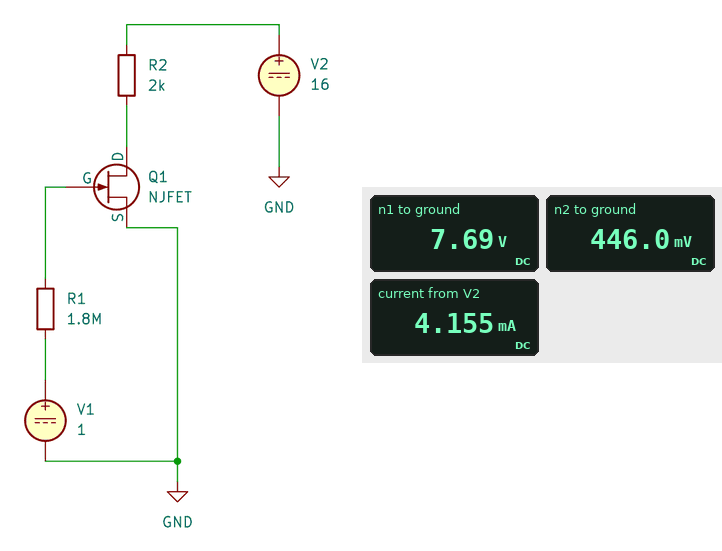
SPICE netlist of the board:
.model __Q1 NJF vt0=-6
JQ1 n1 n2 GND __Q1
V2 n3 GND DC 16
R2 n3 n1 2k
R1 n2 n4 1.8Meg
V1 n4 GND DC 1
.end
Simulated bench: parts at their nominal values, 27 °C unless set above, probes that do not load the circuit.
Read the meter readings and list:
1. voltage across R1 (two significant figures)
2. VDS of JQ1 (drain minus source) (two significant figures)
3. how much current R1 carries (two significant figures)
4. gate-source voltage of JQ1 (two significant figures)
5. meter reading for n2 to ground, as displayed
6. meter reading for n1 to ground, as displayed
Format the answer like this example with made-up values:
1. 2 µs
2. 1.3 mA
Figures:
1. 550 mV
2. 7.7 V
3. 310 nA
4. 450 mV
5. 446.0 mV
6. 7.69 V
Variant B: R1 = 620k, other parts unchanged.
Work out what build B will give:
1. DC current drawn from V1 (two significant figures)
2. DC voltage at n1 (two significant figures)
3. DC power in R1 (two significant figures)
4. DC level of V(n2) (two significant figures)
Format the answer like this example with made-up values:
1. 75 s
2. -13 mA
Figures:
1. 850 nA
2. 7.6 V
3. 450 nW
4. 470 mV
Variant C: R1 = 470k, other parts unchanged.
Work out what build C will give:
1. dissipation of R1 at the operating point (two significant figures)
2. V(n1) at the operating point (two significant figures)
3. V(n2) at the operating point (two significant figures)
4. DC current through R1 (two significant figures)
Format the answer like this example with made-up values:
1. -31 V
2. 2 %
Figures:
1. 580 nW
2. 7.6 V
3. 480 mV
4. 1.1 µA
